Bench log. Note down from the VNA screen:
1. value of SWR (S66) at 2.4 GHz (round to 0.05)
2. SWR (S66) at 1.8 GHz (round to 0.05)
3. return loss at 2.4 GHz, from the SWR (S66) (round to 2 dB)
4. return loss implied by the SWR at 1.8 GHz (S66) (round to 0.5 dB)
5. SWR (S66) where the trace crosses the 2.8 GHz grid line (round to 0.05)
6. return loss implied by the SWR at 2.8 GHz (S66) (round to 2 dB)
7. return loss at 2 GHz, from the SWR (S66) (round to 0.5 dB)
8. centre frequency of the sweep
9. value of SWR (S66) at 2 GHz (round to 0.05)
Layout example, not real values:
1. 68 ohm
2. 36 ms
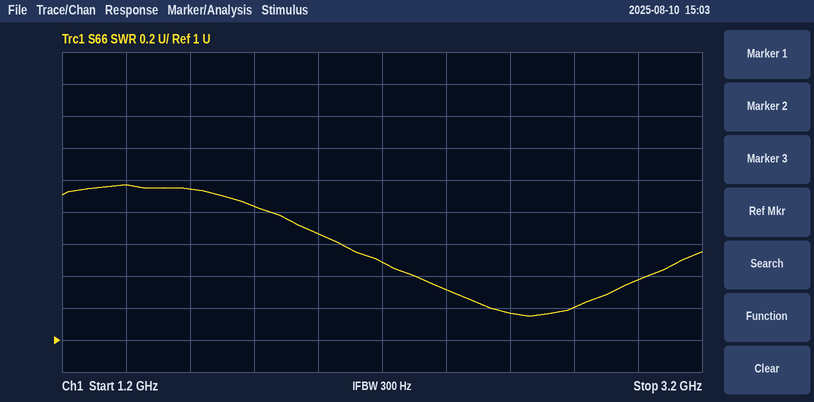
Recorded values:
1. 1.30
2. 1.85
3. 18 dB
4. 10.5 dB
5. 1.20
6. 20 dB
7. 12.0 dB
8. 2.2 GHz
9. 1.65
